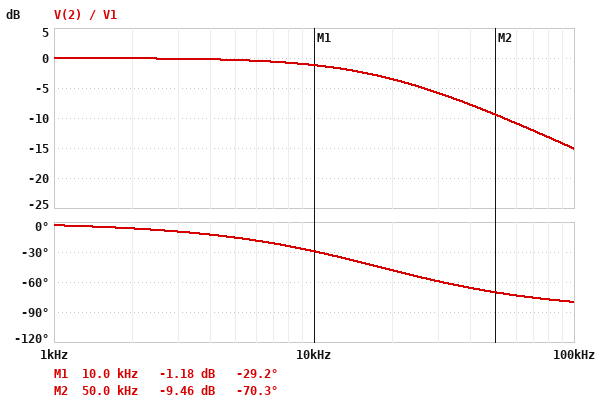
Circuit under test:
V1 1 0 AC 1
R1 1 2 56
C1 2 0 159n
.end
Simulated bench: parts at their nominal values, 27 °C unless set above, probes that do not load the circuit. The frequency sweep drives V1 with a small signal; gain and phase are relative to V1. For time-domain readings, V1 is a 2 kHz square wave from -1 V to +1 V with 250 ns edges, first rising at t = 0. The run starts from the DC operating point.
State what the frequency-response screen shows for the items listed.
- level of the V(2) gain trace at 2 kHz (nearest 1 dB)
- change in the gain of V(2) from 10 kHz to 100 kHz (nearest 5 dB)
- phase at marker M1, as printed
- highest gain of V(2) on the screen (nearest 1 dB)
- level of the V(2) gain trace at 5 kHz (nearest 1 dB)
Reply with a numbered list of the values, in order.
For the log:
1. 0 dB
2. -15 dB
3. -29.2 deg
4. 0 dB
5. 0 dB
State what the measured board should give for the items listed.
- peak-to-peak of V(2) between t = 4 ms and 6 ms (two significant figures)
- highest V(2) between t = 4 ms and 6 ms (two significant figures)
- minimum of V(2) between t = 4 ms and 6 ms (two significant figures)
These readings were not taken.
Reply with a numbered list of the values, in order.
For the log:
1. 2.0 V
2. 1.0 V
3. -1.0 V
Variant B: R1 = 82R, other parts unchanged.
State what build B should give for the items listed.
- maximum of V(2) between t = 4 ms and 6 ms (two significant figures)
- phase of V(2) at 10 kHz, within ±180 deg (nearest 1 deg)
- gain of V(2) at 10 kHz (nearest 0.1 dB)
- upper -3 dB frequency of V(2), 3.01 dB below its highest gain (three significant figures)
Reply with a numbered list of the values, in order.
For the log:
1. 1.0 V
2. -39 deg
3. -2.2 dB
4. 12.2 kHz
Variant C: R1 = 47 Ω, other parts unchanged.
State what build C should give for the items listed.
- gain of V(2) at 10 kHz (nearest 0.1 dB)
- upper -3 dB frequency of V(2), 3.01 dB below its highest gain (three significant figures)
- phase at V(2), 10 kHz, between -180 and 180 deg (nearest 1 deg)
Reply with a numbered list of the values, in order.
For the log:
1. -0.9 dB
2. 21.3 kHz
3. -25 deg
